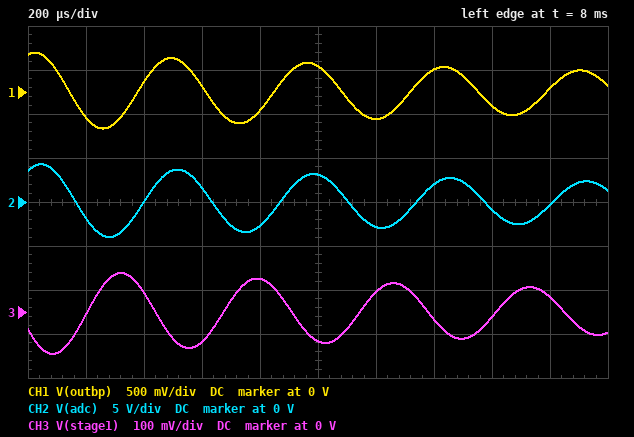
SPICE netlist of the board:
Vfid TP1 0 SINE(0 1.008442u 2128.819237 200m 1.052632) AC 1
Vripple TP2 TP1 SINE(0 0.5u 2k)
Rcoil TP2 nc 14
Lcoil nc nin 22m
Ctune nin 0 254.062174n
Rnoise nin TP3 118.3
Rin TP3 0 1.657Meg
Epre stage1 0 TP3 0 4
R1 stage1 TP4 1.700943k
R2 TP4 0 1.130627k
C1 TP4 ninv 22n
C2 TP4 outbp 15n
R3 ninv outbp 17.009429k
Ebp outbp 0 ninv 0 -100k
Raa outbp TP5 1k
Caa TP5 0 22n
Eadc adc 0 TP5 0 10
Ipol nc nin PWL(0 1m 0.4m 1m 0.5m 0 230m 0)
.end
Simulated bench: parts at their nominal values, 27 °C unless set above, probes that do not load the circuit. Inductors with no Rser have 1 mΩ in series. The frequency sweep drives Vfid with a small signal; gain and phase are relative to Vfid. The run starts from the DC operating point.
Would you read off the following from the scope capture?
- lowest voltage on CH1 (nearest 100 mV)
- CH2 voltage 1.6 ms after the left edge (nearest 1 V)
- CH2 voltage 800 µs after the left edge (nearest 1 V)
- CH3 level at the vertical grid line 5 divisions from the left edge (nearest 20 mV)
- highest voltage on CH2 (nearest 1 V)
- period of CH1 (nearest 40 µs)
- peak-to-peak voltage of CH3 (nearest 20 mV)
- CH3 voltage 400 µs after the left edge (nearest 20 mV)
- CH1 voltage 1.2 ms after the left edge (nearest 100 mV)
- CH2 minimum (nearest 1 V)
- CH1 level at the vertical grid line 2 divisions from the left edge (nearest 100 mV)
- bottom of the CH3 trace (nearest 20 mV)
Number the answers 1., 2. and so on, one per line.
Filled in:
1. -400 mV
2. -1 V
3. -3 V
4. -60 mV
5. 4 V
6. 480 µs
7. 180 mV
8. 40 mV
9. -300 mV
10. -4 V
11. 100 mV
12. -100 mV
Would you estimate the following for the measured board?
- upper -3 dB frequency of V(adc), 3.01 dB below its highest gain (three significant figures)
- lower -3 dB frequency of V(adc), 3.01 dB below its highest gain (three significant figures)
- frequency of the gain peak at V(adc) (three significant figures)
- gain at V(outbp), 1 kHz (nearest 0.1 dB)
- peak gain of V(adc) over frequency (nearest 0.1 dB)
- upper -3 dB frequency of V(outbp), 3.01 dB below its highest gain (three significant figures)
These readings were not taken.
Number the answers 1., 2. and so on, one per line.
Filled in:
1. 2.18 kHz
2. 2.08 kHz
3. 2.13 kHz
4. 14.9 dB
5. 70.8 dB
6. 2.18 kHz
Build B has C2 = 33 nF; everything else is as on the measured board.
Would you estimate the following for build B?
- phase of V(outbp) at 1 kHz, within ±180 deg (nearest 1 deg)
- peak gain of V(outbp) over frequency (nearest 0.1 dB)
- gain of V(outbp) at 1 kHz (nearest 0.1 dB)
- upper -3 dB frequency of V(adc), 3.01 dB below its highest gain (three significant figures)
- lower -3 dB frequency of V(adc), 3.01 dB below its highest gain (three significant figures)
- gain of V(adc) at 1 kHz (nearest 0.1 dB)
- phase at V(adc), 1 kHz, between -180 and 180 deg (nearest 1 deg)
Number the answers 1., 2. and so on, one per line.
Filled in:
1. -111 deg
2. 47.5 dB
3. 16.6 dB
4. 2.17 kHz
5. 2.07 kHz
6. 36.6 dB
7. -119 deg
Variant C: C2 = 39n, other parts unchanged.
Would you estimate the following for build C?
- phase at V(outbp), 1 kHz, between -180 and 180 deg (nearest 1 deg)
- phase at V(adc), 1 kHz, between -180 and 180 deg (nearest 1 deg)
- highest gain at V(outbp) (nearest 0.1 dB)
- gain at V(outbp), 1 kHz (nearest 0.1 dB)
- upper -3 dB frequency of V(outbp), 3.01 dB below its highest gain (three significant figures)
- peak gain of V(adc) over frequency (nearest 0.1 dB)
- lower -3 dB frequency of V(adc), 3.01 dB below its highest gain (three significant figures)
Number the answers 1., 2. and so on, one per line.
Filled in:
1. -115 deg
2. -123 deg
3. 44.9 dB
4. 17.2 dB
5. 2.17 kHz
6. 64.6 dB
7. 2.07 kHz
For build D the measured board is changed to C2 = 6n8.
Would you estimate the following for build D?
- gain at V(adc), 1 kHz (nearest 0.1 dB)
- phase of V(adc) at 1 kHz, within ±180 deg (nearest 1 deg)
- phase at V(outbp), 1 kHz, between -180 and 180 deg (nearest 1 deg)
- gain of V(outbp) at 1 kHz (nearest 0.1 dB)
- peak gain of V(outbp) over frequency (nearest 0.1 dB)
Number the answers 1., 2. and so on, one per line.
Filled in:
1. 34.1 dB
2. -107 deg
3. -99 deg
4. 14.2 dB
5. 47.1 dB
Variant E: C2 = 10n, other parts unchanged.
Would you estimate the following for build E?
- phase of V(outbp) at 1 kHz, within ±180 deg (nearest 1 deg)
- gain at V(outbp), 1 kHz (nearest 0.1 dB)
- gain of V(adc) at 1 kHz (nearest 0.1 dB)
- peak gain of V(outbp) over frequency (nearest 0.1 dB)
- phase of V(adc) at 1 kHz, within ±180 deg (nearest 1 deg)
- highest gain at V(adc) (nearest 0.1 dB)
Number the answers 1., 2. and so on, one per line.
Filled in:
1. -100 deg
2. 14.5 dB
3. 34.4 dB
4. 48.7 dB
5. -108 deg
6. 68.3 dB
